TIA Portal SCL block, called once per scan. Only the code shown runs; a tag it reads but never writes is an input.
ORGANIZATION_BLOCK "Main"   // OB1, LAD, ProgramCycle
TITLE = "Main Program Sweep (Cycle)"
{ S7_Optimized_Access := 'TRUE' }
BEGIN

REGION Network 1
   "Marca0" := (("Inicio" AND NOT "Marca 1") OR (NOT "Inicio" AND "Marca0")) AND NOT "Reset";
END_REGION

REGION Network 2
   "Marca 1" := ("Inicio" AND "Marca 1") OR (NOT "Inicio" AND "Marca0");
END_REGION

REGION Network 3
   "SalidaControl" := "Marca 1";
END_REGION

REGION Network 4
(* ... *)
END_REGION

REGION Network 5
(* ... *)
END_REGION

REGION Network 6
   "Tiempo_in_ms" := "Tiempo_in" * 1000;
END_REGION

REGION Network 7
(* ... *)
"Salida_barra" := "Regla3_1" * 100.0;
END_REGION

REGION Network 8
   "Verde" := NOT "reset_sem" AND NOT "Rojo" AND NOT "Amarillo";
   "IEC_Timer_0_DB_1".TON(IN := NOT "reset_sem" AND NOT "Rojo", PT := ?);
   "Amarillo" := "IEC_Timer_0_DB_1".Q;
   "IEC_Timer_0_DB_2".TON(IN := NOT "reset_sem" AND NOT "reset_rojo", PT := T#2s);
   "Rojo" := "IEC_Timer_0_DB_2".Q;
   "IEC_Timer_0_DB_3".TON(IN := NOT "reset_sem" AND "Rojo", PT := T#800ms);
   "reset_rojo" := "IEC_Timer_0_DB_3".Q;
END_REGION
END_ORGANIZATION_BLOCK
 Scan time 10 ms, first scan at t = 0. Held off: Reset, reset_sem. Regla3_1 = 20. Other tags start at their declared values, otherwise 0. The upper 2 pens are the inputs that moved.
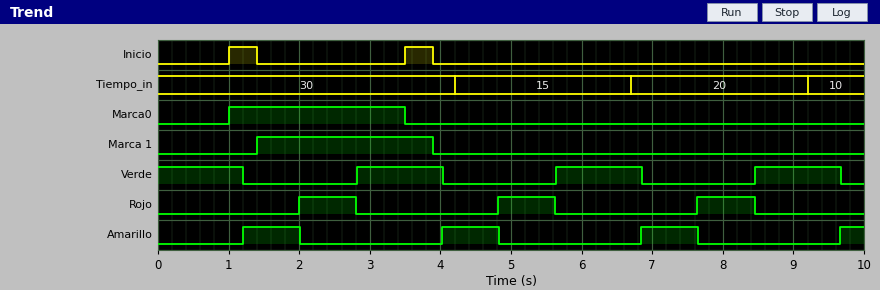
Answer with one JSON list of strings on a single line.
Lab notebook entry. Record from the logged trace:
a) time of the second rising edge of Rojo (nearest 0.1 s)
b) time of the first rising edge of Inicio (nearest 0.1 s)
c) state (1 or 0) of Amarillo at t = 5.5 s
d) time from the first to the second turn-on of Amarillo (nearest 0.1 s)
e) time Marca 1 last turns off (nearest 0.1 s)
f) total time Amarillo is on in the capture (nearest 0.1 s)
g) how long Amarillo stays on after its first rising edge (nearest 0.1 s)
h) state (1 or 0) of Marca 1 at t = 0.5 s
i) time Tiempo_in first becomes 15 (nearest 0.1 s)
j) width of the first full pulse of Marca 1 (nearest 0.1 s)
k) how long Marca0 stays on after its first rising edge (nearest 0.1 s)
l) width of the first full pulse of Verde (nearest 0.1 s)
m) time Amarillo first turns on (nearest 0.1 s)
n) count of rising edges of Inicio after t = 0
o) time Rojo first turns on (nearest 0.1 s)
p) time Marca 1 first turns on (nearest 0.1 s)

["4.8 s", "1.0 s", "0", "2.8 s", "3.9 s", "2.8 s", "0.8 s", "0", "4.2 s", "2.5 s", "2.5 s", "1.2 s", "1.2 s", "2", "2.0 s", "1.4 s"]
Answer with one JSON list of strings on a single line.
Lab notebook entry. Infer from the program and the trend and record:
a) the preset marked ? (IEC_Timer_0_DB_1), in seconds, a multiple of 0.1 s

["1.2 s"]
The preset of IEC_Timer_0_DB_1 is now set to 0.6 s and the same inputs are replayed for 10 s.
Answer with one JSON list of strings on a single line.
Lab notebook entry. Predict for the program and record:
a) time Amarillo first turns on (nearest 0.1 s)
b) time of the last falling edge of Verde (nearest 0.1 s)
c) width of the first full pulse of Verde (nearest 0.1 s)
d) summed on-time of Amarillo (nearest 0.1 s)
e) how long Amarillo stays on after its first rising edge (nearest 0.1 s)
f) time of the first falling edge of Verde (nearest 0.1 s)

["0.6 s", "9.1 s", "0.6 s", "5.2 s", "1.4 s", "0.6 s"]
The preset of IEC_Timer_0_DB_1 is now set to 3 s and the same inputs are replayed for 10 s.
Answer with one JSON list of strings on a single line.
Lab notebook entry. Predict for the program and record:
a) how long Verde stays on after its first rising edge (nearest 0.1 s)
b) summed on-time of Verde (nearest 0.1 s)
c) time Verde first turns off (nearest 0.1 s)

["2.0 s", "7.6 s", "2.0 s"]
